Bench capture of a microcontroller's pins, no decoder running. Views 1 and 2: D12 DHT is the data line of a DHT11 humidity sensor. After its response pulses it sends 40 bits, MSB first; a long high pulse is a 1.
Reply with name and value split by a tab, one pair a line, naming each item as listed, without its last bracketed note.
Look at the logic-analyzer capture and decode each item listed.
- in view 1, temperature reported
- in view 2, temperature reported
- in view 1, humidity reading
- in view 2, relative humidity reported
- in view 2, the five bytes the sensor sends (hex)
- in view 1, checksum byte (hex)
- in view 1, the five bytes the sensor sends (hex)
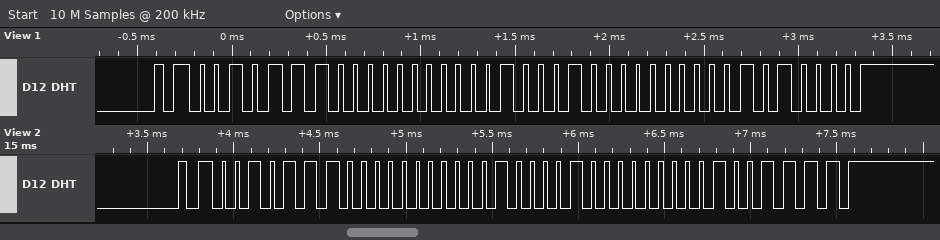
in view 1, temperature reported	34.0 °C
in view 2, temperature reported	33.0 °C
in view 1, humidity reading	46 %
in view 2, relative humidity reported	46 %
in view 2, the five bytes the sensor sends	2E 00 21 00 4F
in view 1, checksum byte	0x50
in view 1, the five bytes the sensor sends	2E 00 22 00 50
